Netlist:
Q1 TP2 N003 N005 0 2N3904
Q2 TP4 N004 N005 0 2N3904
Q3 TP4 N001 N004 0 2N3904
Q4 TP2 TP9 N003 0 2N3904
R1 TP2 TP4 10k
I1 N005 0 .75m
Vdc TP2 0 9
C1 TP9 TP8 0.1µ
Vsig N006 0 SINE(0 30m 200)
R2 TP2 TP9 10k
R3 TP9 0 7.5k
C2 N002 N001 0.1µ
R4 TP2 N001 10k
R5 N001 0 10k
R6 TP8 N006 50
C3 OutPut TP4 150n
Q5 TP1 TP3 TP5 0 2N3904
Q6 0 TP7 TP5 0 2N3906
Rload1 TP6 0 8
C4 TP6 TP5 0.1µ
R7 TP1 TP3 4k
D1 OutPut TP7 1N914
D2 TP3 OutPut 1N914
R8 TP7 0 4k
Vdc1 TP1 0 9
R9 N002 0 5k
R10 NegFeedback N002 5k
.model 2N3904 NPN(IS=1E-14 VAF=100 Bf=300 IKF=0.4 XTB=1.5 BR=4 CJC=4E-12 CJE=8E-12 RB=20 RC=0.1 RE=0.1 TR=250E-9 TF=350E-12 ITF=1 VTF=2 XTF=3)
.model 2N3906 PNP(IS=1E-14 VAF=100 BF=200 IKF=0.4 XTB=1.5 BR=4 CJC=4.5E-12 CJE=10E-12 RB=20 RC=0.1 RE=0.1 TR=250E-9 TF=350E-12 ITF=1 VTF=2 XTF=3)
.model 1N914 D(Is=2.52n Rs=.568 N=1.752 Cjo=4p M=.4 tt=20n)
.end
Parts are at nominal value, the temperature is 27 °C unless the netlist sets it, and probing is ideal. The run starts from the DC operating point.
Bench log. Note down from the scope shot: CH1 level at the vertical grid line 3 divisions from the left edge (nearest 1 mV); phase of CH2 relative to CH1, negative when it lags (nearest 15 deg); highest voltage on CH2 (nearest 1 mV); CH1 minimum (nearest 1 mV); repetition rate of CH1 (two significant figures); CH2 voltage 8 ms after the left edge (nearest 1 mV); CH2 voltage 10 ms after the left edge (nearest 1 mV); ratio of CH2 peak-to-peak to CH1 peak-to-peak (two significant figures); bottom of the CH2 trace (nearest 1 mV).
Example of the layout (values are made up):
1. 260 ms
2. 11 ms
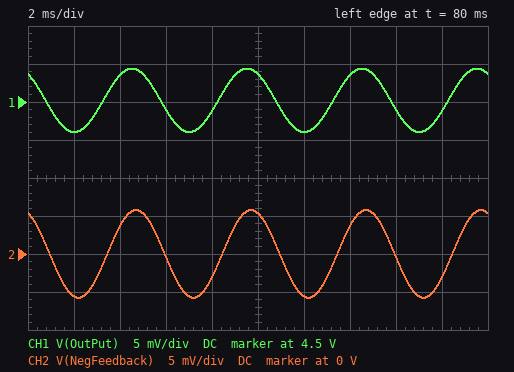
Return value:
1. 4.499 V
2. -15 deg
3. 6 mV
4. 4.496 V
5. 200 Hz
6. -3 mV
7. 5 mV
8. 1.4
9. -6 mV
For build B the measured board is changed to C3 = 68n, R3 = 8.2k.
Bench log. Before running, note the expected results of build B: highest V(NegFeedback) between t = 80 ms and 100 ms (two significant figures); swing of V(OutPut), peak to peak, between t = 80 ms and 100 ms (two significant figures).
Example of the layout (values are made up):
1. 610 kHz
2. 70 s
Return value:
1. 6.1 mV
2. 4.5 mV
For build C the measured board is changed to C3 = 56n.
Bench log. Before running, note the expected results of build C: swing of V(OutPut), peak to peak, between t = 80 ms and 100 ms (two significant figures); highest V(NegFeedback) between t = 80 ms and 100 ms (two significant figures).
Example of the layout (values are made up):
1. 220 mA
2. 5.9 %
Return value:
1. 3.4 mV
2. 5.9 mV
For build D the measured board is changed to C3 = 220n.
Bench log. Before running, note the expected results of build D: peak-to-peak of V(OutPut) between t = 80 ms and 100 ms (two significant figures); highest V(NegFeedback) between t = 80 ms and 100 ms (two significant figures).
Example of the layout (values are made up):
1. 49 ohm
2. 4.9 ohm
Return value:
1. 11 mV
2. 5.6 mV
